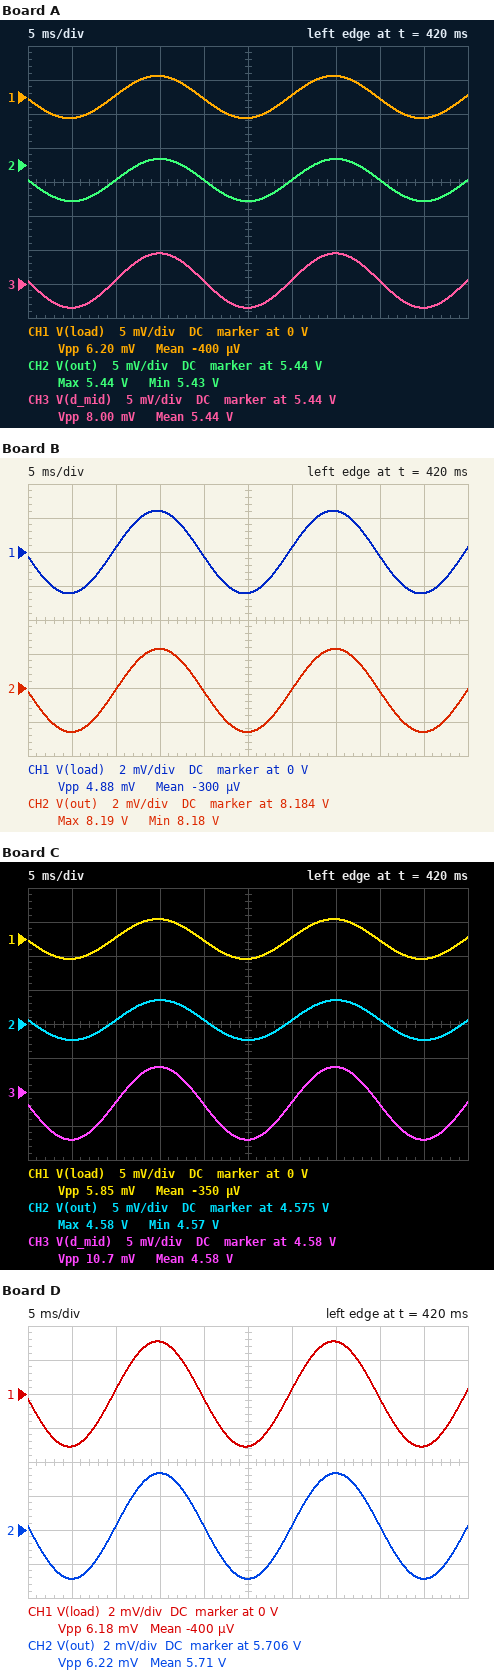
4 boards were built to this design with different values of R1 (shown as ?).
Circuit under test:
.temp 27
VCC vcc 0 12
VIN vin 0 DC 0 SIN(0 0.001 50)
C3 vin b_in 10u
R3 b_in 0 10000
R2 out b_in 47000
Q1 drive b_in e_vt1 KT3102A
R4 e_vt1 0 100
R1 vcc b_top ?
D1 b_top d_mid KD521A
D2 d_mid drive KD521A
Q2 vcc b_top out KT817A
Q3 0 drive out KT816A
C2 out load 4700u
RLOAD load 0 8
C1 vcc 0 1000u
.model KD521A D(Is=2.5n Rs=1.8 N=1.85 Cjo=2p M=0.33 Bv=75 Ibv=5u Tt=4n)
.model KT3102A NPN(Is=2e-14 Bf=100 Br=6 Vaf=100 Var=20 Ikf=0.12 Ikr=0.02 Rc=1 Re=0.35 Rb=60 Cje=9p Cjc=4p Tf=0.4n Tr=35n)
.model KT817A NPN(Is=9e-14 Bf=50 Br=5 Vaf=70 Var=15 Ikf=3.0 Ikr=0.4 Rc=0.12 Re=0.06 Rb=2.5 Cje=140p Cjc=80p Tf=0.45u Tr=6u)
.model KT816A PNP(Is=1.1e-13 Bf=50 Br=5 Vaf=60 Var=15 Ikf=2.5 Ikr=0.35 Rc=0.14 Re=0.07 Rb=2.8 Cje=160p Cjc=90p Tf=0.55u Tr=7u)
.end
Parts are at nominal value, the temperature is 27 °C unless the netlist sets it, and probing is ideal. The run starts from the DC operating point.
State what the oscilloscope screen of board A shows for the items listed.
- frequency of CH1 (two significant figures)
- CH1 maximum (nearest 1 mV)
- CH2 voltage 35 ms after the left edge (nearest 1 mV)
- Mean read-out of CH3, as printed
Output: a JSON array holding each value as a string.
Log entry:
["50 Hz", "3 mV", "5.441 V", "5.44 V"]
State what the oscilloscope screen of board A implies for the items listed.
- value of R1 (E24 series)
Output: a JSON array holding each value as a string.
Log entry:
["3.6 kΩ"]
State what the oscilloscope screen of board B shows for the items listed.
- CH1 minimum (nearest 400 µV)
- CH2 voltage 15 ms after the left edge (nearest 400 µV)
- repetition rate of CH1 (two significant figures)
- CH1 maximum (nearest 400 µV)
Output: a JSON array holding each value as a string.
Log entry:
["-2.4 mV", "8.1864 V", "50 Hz", "2.4 mV"]
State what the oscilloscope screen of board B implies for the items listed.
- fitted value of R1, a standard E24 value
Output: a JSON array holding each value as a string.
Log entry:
["750 Ω"]
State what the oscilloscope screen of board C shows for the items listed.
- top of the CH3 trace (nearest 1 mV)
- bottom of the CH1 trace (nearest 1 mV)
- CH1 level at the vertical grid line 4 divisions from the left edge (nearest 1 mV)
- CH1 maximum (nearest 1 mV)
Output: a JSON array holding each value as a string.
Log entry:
["4.584 V", "-3 mV", "0 V", "3 mV"]
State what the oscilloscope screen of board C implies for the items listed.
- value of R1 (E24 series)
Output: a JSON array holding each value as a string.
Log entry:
["7.5 kΩ"]
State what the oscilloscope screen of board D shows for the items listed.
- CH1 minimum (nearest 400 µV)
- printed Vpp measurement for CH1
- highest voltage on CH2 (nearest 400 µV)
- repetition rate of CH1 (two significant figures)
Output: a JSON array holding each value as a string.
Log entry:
["-3.2 mV", "6.18 mV", "5.7092 V", "50 Hz"]
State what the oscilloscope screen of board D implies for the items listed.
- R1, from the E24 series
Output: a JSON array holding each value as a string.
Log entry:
["3 kΩ"]
